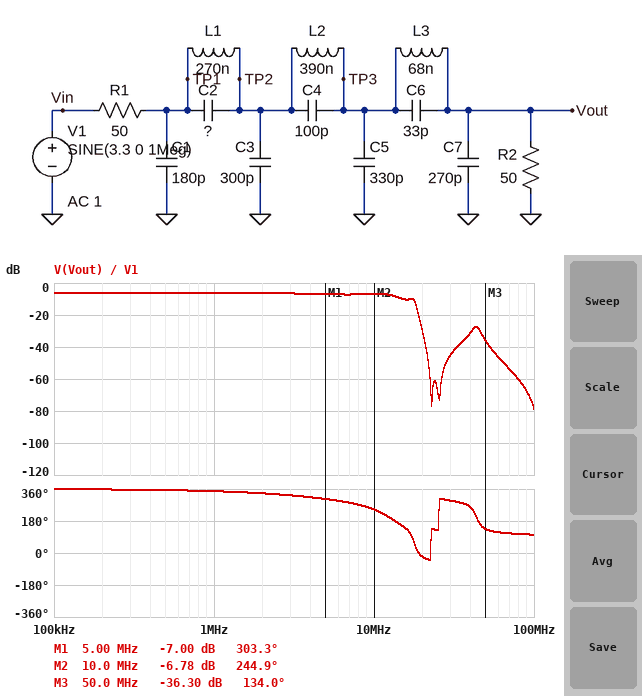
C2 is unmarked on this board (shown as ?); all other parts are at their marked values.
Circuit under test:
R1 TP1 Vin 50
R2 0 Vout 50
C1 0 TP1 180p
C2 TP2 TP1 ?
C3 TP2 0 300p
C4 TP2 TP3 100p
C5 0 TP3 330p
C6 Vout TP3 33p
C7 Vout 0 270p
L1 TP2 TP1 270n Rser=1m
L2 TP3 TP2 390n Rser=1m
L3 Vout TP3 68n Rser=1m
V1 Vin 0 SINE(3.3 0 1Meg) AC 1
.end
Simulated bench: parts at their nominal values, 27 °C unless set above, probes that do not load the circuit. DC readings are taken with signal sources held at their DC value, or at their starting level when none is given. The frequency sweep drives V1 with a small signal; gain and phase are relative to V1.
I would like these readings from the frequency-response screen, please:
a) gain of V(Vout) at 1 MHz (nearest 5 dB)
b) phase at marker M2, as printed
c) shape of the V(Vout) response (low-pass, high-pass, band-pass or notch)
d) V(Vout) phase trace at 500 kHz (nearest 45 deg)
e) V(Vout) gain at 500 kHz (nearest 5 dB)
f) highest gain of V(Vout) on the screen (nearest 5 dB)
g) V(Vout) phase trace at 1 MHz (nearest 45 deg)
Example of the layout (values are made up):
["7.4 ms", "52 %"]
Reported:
["-5 dB", "244.9 deg", "low-pass", "360 deg", "-5 dB", "-5 dB", "360 deg"]
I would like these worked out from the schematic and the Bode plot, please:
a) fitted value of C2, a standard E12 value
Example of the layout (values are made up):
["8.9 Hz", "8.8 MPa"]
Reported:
["180 pF"]
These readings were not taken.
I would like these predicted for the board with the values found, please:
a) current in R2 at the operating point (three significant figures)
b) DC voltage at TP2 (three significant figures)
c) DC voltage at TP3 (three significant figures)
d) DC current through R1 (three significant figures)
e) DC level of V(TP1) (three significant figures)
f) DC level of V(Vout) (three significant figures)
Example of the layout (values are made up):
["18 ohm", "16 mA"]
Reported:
["33.0 mA", "1.65 V", "1.65 V", "33.0 mA", "1.65 V", "1.65 V"]
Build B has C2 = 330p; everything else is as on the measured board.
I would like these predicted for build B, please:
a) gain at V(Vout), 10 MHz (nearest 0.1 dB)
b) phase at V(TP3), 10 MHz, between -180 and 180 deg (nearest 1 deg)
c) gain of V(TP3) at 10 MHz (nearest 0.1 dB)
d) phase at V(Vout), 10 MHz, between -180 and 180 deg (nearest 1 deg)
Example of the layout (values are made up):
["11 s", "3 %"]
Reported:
["-6.9 dB", "-115 deg", "-7.5 dB", "-120 deg"]
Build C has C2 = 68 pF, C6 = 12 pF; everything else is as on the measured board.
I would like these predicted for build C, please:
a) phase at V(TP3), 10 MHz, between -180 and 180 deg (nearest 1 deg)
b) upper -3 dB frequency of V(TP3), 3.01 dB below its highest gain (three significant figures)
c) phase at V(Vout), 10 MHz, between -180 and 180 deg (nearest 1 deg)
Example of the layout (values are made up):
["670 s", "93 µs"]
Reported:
["-107 deg", "13.4 MHz", "-112 deg"]
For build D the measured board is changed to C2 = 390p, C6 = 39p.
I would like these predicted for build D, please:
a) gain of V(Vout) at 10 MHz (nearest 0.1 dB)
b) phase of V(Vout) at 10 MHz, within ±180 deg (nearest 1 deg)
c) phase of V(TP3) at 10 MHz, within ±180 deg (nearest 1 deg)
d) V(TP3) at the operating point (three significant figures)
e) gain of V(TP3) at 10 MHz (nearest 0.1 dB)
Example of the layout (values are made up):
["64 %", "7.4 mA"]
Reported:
["-7.0 dB", "-123 deg", "-118 deg", "1.65 V", "-7.6 dB"]
